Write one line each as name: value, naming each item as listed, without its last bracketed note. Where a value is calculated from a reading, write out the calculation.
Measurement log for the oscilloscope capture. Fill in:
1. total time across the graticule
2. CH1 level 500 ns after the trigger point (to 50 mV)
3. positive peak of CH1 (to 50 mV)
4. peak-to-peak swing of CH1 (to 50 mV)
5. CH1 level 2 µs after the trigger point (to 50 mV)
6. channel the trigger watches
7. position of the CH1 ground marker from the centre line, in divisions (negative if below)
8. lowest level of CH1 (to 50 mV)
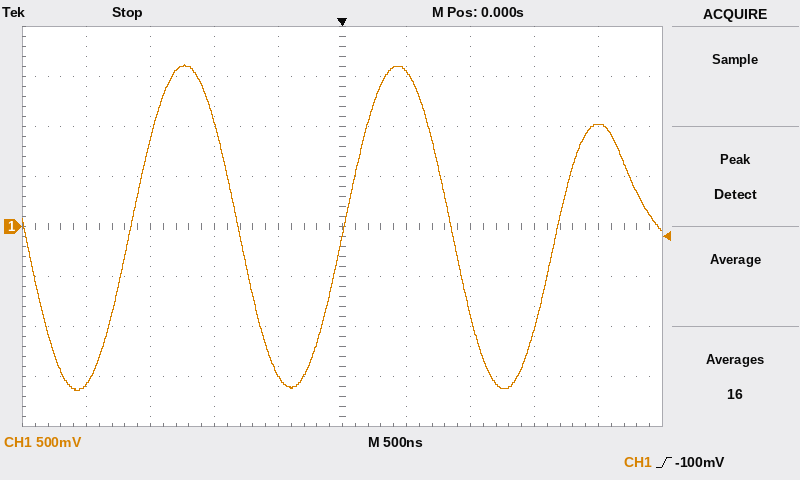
total time across the graticule: 5 µs
CH1 level 500 ns after the trigger point: 1.55 V
positive peak of CH1: 1.60 V
peak-to-peak swing of CH1: 1.60 V − (-1.65 V) = 3.25 V
CH1 level 2 µs after the trigger point: 1.00 V
channel the trigger watches: CH1
position of the CH1 ground marker from the centre line, in divisions: 0.0 div
lowest level of CH1: -1.65 V
